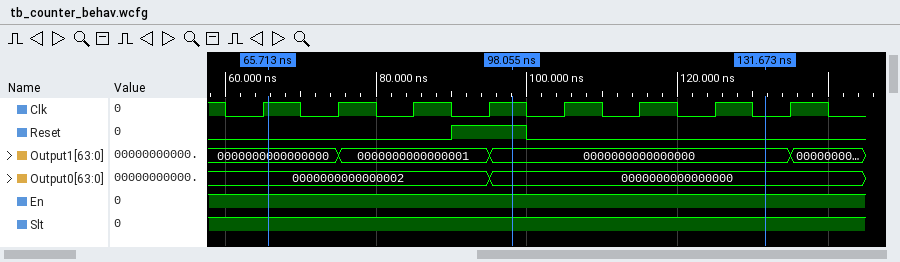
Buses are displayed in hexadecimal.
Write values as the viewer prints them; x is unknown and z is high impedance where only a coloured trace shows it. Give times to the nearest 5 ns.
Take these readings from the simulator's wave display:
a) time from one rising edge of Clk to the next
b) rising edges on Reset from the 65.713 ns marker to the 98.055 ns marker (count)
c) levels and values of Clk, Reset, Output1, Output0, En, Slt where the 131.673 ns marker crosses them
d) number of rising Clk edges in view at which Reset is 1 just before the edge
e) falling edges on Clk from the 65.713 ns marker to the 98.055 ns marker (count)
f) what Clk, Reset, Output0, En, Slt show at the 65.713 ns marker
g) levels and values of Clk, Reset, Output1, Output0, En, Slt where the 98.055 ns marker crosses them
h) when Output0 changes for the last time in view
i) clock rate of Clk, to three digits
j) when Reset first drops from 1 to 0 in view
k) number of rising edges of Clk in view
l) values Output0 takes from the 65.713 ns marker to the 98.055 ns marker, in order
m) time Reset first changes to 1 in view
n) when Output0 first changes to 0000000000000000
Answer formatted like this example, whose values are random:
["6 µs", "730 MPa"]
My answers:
["10 ns", "1", "Clk=0, Reset=0, Output1=0000000000000000, Output0=0000000000000000, En=1, Slt=1", "1", "3", "Clk=1, Reset=0, Output0=0000000000000002, En=1, Slt=1", "Clk=1, Reset=1, Output1=0000000000000000, Output0=0000000000000000, En=1, Slt=1", "95 ns", "100 MHz", "100 ns", "8", "0000000000000002, 0000000000000000", "90 ns", "95 ns"]
